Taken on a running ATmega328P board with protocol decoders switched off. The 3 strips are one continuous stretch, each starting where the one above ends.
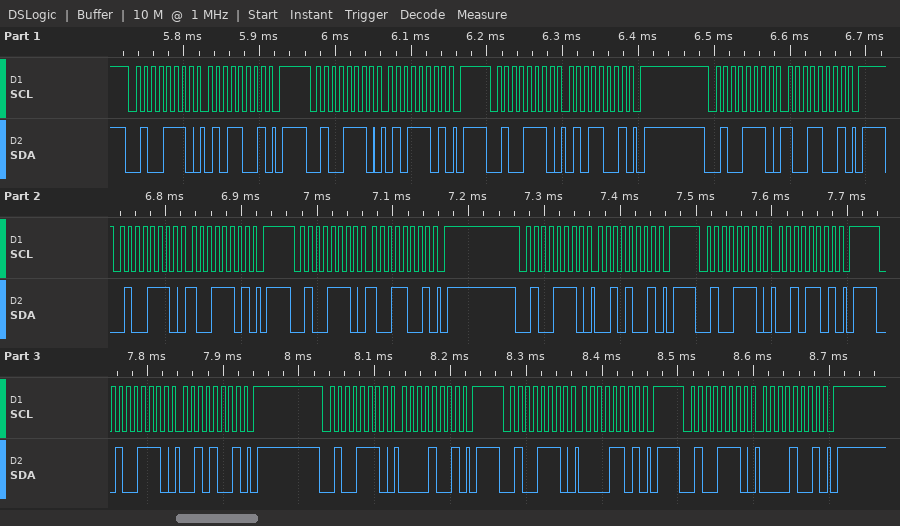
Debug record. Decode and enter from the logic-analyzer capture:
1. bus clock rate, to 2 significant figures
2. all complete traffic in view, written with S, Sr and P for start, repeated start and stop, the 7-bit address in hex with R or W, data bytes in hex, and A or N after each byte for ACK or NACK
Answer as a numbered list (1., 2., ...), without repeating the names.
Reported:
1. 100 kHz
2. S 27W A 59 A P S 27W A 5D A P S 27W A 59 A P S 27W A 99 A P S 27W A 9D A P S 27W A 99 A P S 27W A 29 A P S 27W A 2D A P S 27W A 29 A P S 27W A 09 A P S 27W A 0D A P S 27W A 09 A P
